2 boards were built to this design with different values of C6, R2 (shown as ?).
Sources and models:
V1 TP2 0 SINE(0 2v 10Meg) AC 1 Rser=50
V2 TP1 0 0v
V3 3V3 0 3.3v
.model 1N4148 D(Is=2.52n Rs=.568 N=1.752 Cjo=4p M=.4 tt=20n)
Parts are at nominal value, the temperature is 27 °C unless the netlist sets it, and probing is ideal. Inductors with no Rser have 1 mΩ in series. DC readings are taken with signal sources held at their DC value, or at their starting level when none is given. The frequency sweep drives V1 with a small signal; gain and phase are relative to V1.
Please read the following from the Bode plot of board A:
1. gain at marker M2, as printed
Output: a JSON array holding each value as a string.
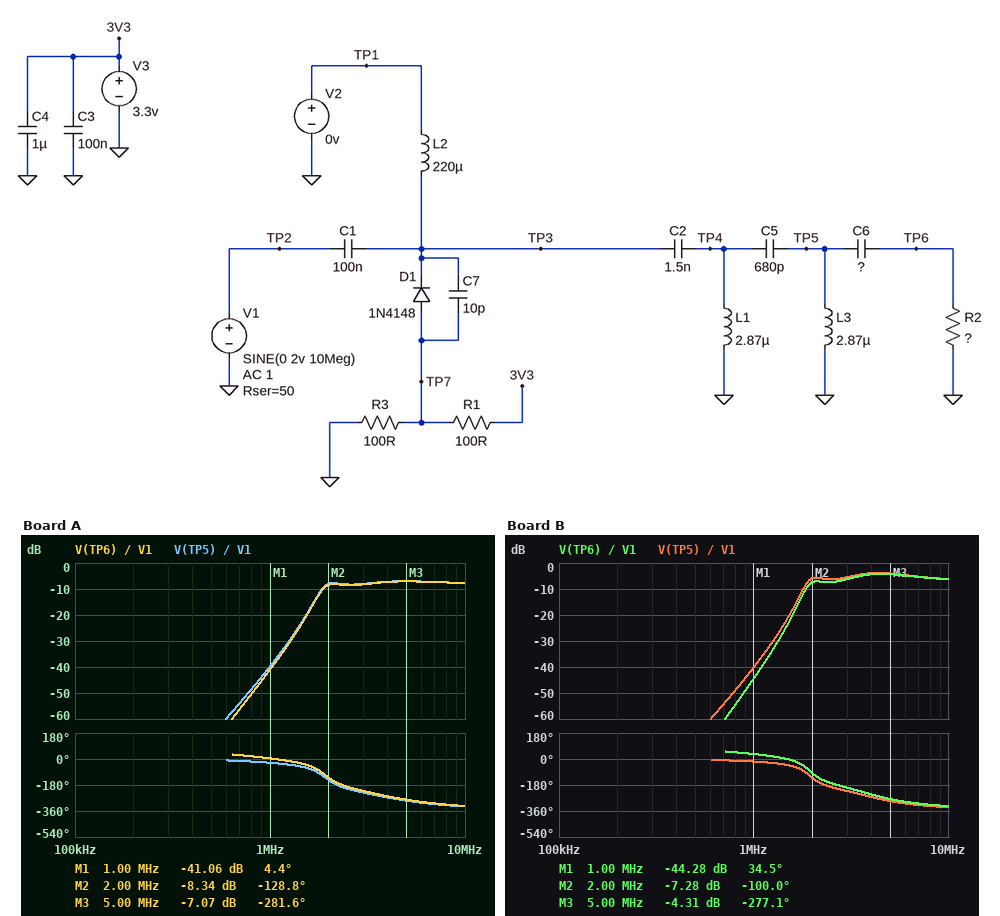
["-8.34 dB"]
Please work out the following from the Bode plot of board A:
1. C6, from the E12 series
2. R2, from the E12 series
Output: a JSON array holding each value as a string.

["3.3 nF", "82 Ω"]
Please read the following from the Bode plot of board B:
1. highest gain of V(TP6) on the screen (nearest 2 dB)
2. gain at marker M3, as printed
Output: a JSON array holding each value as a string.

["-4 dB", "-4.31 dB"]
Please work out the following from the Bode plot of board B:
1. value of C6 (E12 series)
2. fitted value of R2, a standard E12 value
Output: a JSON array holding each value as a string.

["820 pF", "150 Ω"]
